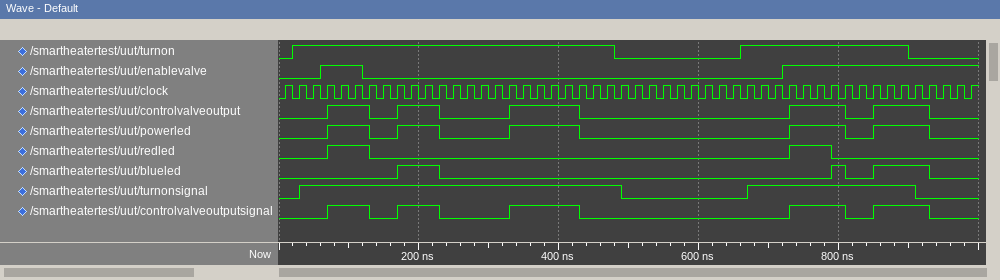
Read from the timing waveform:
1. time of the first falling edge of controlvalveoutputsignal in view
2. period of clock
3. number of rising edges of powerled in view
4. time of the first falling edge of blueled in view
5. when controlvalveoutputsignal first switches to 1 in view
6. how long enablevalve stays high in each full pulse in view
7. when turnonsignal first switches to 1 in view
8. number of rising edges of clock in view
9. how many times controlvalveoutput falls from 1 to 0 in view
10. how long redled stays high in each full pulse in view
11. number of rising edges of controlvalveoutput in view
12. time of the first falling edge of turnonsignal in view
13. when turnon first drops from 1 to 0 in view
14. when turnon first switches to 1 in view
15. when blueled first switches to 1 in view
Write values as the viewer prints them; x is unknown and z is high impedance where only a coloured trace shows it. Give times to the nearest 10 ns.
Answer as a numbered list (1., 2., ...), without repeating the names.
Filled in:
1. 130 ns
2. 20 ns
3. 5
4. 230 ns
5. 70 ns
6. 60 ns
7. 30 ns
8. 50
9. 5
10. 60 ns, 60 ns
11. 5
12. 490 ns
13. 480 ns
14. 20 ns
15. 170 ns
